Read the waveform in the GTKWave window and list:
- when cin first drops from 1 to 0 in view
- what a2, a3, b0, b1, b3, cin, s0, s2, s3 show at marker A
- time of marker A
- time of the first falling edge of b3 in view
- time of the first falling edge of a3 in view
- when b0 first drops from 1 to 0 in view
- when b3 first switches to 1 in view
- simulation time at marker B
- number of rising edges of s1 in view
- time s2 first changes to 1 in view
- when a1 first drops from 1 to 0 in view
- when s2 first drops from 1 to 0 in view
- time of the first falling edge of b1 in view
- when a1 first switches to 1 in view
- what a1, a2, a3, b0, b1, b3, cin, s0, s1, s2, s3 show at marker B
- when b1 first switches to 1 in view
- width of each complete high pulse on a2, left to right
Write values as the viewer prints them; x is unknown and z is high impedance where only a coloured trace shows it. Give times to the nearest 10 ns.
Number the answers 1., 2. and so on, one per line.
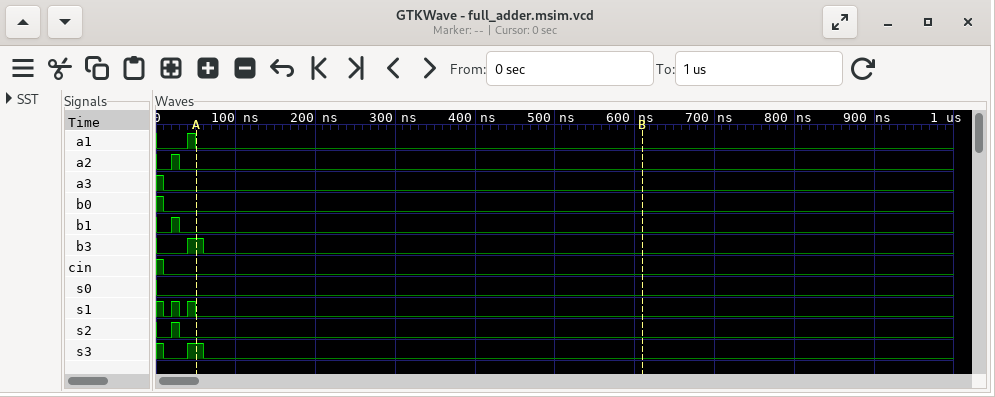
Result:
1. 10 ns
2. a2=0, a3=0, b0=0, b1=0, b3=1, cin=0, s0=0, s2=0, s3=1
3. 50 ns
4. 60 ns
5. 10 ns
6. 10 ns
7. 40 ns
8. 610 ns
9. 2
10. 20 ns
11. 50 ns
12. 30 ns
13. 30 ns
14. 40 ns
15. a1=0, a2=0, a3=0, b0=0, b1=0, b3=0, cin=0, s0=0, s1=0, s2=0, s3=0
16. 20 ns
17. 10 ns
